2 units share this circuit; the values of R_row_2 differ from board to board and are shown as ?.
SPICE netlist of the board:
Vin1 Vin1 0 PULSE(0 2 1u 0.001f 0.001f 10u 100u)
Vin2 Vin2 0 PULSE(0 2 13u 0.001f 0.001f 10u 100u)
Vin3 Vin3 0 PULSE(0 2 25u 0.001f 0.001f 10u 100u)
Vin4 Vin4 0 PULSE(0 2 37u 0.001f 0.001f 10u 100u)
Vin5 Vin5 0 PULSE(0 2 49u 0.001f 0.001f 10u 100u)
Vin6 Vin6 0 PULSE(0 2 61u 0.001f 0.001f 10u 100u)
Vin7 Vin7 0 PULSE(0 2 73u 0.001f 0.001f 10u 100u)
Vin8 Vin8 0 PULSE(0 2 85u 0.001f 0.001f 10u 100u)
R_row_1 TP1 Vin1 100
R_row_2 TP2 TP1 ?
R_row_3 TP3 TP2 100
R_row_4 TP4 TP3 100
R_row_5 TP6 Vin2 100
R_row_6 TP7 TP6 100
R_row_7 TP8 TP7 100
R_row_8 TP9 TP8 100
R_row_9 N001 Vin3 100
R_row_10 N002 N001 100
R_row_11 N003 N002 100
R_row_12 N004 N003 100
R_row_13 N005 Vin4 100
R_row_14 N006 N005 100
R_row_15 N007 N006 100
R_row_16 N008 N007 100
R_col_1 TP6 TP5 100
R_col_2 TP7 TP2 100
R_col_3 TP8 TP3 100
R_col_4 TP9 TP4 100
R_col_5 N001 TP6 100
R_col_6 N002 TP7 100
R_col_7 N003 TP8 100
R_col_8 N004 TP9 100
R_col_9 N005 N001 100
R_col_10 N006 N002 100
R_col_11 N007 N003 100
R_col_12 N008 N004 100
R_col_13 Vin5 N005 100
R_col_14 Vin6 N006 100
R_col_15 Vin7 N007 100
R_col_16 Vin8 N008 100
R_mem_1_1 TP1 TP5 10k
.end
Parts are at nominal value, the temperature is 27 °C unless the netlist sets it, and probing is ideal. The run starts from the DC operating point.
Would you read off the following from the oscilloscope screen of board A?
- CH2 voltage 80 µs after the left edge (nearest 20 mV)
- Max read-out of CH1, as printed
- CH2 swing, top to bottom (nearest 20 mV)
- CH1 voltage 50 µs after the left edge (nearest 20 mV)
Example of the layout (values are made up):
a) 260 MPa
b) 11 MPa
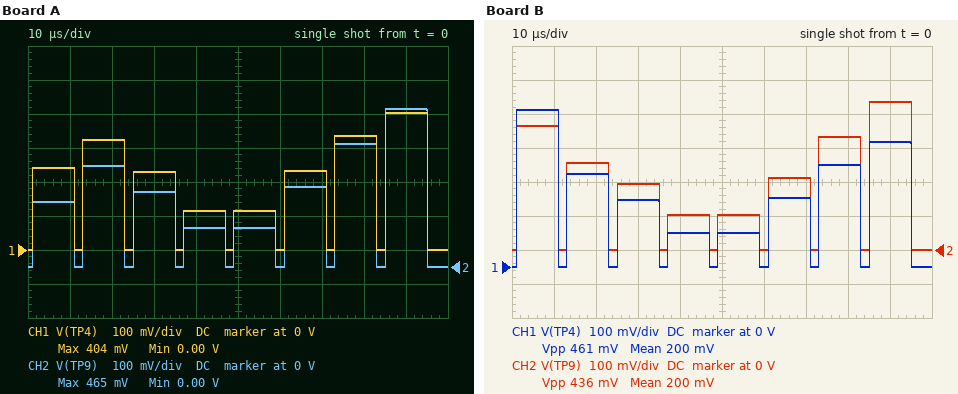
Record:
a) 360 mV
b) 404 mV
c) 460 mV
d) 120 mV
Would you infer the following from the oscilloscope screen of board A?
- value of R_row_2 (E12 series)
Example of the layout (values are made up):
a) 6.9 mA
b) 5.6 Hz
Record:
a) 330 Ω
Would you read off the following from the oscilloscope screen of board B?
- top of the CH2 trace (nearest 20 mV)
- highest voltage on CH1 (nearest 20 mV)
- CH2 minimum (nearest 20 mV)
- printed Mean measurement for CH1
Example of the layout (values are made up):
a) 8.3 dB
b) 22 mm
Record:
a) 440 mV
b) 460 mV
c) 0 V
d) 200 mV
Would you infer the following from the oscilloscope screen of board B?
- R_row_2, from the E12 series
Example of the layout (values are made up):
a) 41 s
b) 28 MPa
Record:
a) 68 Ω
